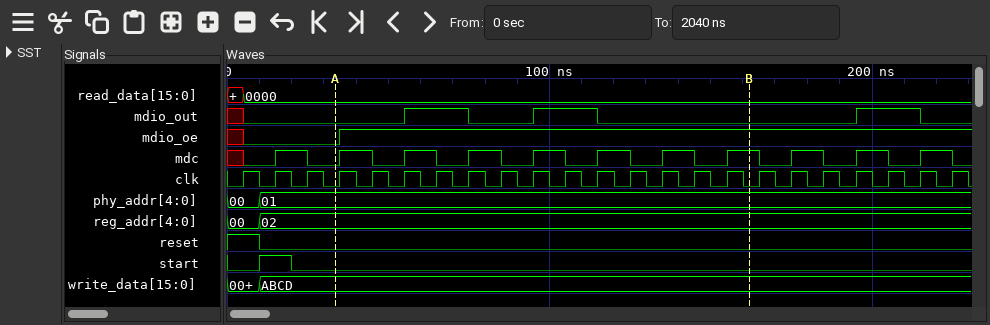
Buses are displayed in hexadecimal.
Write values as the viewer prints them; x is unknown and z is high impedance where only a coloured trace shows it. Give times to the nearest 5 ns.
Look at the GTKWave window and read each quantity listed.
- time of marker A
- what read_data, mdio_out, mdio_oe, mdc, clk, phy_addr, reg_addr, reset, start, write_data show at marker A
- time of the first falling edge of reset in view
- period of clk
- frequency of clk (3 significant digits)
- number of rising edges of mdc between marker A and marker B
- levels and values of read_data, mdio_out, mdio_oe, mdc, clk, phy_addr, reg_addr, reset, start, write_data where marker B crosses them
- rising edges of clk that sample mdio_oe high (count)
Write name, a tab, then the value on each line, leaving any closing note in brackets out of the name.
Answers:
time of marker A	35 ns
what read_data, mdio_out, mdio_oe, mdc, clk, phy_addr, reg_addr, reset, start, write_data show at marker A	read_data=0000, mdio_out=0, mdio_oe=0, mdc=0, clk=0, phy_addr=01, reg_addr=02, reset=0, start=0, write_data=ABCD
time of the first falling edge of reset in view	10 ns
period of clk	10 ns
frequency of clk	100 MHz
number of rising edges of mdc between marker A and marker B	7
levels and values of read_data, mdio_out, mdio_oe, mdc, clk, phy_addr, reg_addr, reset, start, write_data where marker B crosses them	read_data=0000, mdio_out=0, mdio_oe=1, mdc=1, clk=0, phy_addr=01, reg_addr=02, reset=0, start=0, write_data=ABCD
rising edges of clk that sample mdio_oe high	19
